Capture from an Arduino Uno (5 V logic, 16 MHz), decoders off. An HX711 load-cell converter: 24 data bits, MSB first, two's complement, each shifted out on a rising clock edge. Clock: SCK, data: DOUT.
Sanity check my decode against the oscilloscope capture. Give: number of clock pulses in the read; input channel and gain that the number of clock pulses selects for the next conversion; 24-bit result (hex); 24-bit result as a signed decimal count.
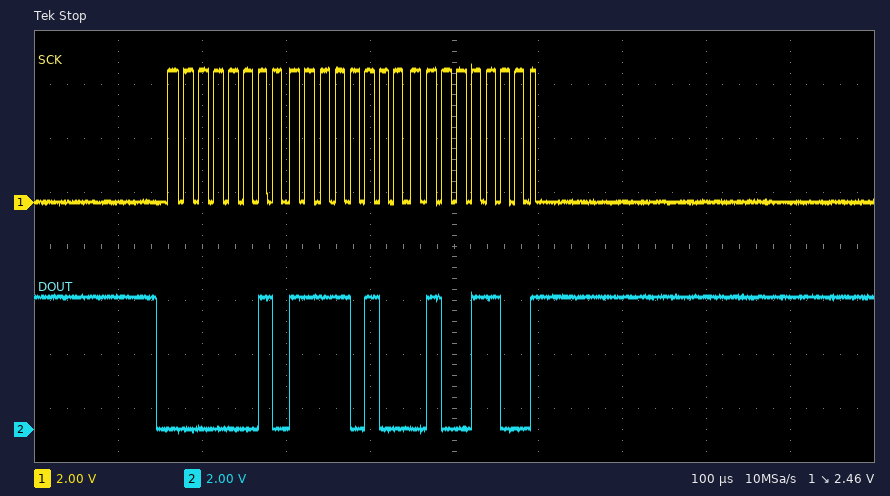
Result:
25
channel A, gain 128
0x02F44C
193612
